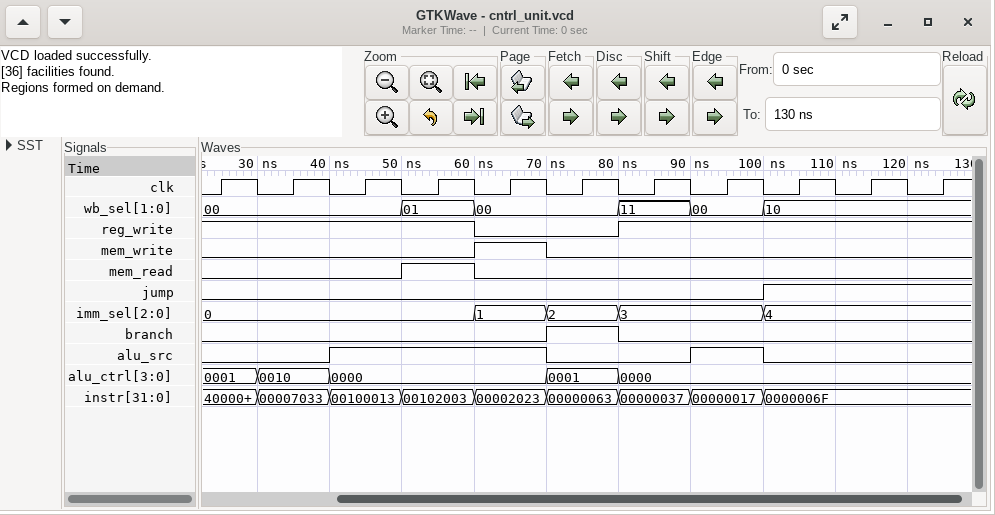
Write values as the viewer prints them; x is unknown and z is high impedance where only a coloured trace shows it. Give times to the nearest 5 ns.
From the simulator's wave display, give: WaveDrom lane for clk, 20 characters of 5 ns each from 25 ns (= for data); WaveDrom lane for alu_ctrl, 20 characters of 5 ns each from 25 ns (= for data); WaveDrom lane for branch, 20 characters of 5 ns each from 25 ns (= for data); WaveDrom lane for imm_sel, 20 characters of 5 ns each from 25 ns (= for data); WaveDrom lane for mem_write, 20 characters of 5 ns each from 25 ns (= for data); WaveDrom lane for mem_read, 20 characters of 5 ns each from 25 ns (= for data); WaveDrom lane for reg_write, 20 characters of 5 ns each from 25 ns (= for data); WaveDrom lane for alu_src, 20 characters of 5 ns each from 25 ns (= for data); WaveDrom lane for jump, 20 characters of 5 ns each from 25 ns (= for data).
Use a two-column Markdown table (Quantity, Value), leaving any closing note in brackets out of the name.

| Quantity | Value |
|---|---|
| WaveDrom lane for clk, 20 characters of 5 ns each from 25 ns | {name: 'clk', wave: '10101010101010101010'} |
| WaveDrom lane for alu_ctrl, 20 characters of 5 ns each from 25 ns | {name: 'alu_ctrl', wave: '==.=.....=.=........', data: '0001 0010 0000 0001 0000'} |
| WaveDrom lane for branch, 20 characters of 5 ns each from 25 ns | {name: 'branch', wave: '0........1.0........'} |
| WaveDrom lane for imm_sel, 20 characters of 5 ns each from 25 ns | {name: 'imm_sel', wave: '=......=.=.=...=....', data: '0 1 2 3 4'} |
| WaveDrom lane for mem_write, 20 characters of 5 ns each from 25 ns | {name: 'mem_write', wave: '0......1.0..........'} |
| WaveDrom lane for mem_read, 20 characters of 5 ns each from 25 ns | {name: 'mem_read', wave: '0....1.0............'} |
| WaveDrom lane for reg_write, 20 characters of 5 ns each from 25 ns | {name: 'reg_write', wave: '1......0...1........'} |
| WaveDrom lane for alu_src, 20 characters of 5 ns each from 25 ns | {name: 'alu_src', wave: '0..1.....0...1.0....'} |
| WaveDrom lane for jump, 20 characters of 5 ns each from 25 ns | {name: 'jump', wave: '0..............1....'} |
